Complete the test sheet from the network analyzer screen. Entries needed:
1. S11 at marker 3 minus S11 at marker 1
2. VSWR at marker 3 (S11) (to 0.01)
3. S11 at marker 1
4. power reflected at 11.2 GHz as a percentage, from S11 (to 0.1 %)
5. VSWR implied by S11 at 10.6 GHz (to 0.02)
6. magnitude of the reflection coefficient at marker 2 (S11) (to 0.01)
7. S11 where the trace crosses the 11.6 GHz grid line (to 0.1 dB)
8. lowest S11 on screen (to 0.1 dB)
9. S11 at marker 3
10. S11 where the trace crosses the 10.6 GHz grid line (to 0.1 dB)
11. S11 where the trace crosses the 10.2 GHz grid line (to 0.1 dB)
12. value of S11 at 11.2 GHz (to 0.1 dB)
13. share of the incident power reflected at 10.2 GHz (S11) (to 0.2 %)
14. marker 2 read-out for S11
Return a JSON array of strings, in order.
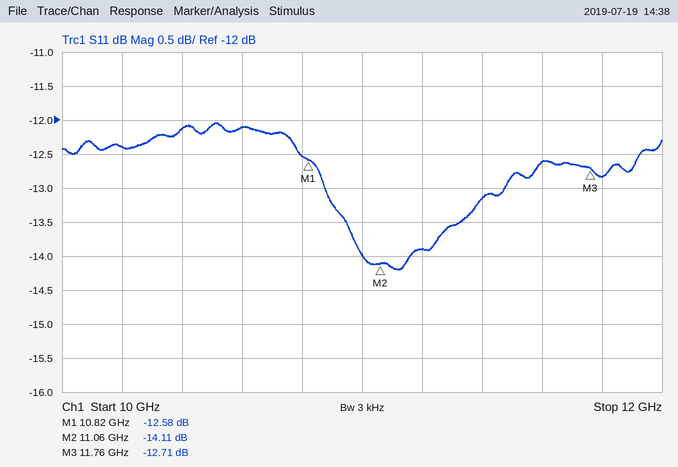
["-0.13 dB", "1.60", "-12.58 dB", "4.1 %", "1.66", "0.20", "-12.6 dB", "-14.2 dB", "-12.71 dB", "-12.1 dB", "-12.4 dB", "-13.9 dB", "5.8 %", "-14.11 dB"]
